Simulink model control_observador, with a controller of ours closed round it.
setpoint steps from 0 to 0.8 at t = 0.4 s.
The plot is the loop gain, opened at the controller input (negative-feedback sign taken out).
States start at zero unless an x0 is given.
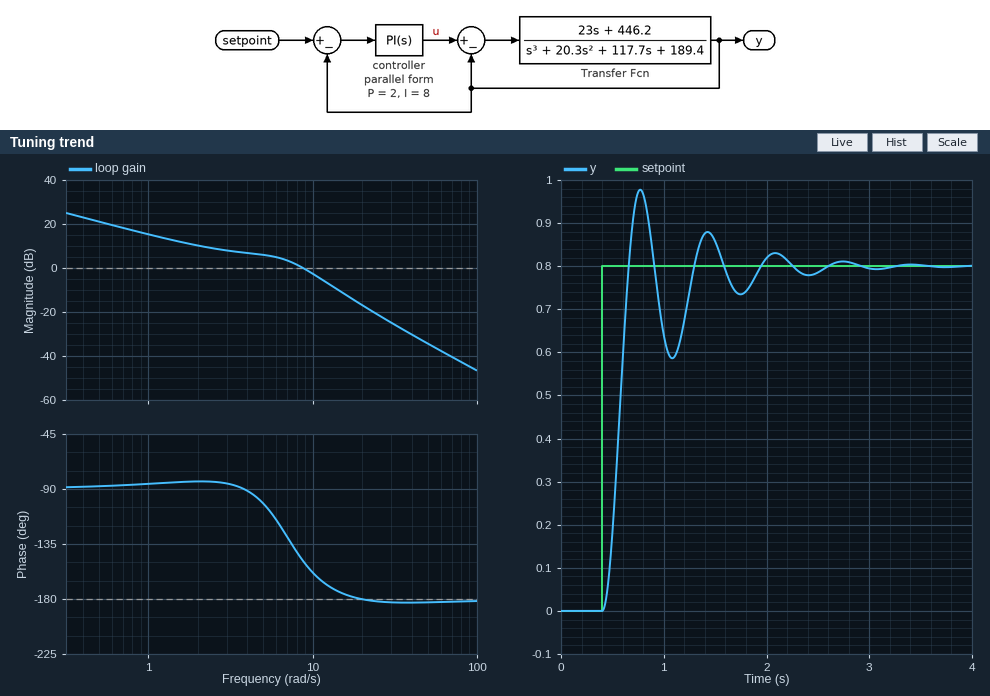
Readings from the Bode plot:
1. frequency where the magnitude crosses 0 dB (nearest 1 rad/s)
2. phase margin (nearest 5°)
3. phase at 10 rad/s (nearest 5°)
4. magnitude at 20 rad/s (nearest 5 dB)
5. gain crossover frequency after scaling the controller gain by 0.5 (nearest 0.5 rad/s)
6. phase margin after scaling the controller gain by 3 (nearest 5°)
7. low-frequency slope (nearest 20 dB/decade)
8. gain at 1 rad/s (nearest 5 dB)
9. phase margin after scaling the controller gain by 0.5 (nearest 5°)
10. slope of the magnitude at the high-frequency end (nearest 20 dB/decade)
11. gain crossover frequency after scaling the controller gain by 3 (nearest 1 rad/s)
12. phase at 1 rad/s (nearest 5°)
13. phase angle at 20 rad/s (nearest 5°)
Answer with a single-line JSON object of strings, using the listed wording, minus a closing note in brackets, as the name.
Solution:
{"frequency where the magnitude crosses 0 dB": "9 rad/s", "phase margin": "30°", "phase at 10 rad/s": "-160°", "magnitude at 20 rad/s": "-15 dB", "gain crossover frequency after scaling the controller gain by 0.5": "5.0 rad/s", "phase margin after scaling the controller gain by 3": "5°", "low-frequency slope": "-20 dB/decade", "gain at 1 rad/s": "15 dB", "phase margin after scaling the controller gain by 0.5": "80°", "slope of the magnitude at the high-frequency end": "-40 dB/decade", "gain crossover frequency after scaling the controller gain by 3": "14 rad/s", "phase at 1 rad/s": "-85°", "phase angle at 20 rad/s": "-180°"}
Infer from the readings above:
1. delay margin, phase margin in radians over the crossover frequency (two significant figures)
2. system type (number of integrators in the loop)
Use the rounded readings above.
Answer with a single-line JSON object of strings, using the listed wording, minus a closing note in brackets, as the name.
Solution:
{"delay margin, phase margin in radians over the crossover frequency": "0.058 s", "system type": "1"}
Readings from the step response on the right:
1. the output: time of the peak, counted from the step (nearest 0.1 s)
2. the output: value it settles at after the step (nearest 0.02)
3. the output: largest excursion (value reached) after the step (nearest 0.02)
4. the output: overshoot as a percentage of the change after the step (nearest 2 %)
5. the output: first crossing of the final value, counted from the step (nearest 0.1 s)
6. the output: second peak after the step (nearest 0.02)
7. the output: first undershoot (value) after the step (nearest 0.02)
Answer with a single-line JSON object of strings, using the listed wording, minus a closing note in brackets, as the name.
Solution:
{"the output: time of the peak, counted from the step": "0.4 s", "the output: value it settles at after the step": "0.80", "the output: largest excursion (value reached) after the step": "0.98", "the output: overshoot as a percentage of the change after the step": "22 %", "the output: first crossing of the final value, counted from the step": "0.3 s", "the output: second peak after the step": "0.88", "the output: first undershoot (value) after the step": "0.58"}
